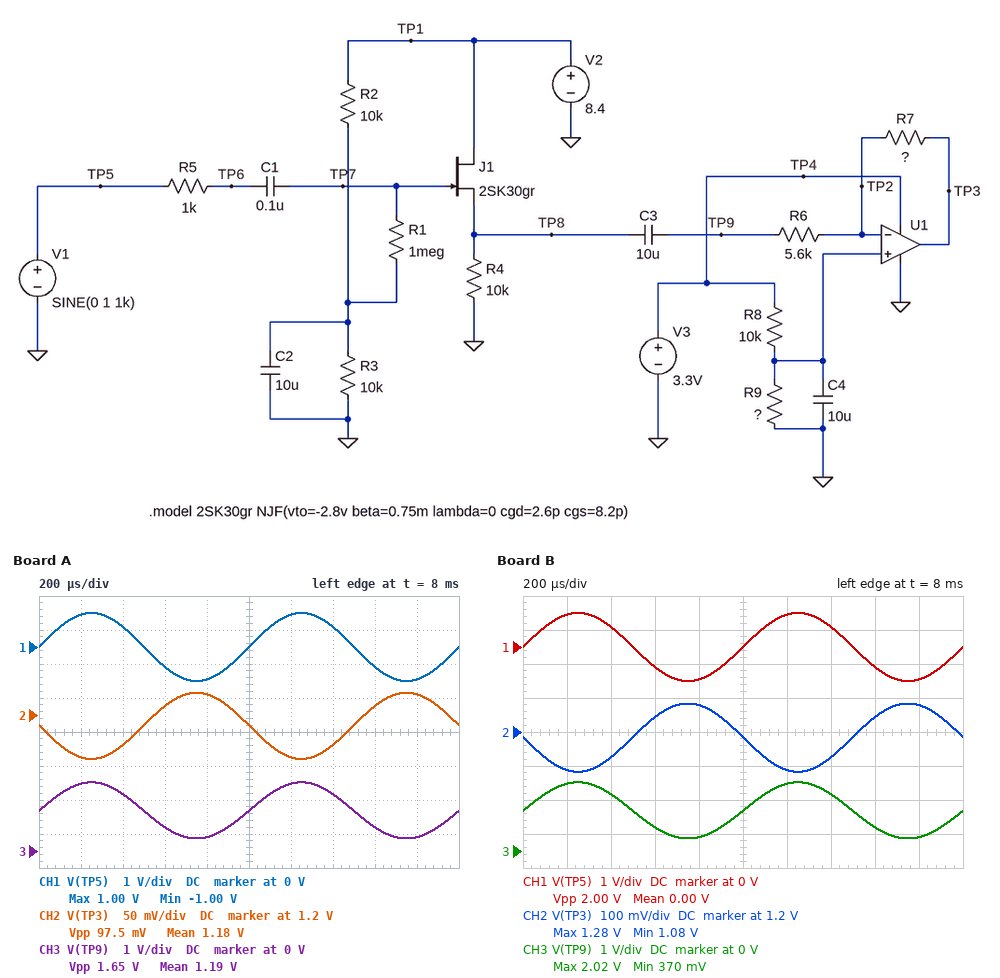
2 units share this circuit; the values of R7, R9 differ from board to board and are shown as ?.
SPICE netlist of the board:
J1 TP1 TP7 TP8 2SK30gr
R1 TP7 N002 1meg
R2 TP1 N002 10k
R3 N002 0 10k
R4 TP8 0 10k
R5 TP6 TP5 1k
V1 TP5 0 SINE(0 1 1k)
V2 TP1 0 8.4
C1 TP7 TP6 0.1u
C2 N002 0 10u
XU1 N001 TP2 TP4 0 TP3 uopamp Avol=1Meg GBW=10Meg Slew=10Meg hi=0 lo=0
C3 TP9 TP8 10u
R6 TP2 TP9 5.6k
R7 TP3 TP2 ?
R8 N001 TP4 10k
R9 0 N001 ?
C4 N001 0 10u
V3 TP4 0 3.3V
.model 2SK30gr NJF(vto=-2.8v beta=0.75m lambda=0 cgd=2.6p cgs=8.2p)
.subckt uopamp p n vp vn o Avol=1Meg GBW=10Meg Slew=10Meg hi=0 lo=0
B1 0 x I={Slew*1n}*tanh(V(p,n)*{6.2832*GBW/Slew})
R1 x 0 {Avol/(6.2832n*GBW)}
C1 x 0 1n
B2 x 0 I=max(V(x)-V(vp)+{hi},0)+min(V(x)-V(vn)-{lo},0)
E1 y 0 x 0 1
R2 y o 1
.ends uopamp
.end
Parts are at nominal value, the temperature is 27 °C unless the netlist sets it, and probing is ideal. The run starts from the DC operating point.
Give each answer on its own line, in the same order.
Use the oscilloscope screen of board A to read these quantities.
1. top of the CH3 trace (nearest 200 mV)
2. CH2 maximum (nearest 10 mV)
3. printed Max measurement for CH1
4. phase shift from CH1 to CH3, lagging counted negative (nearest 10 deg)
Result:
2.0 V
1.23 V
1.00 V
0 deg
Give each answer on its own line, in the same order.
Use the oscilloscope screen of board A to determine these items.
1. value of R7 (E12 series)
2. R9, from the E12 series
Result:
330 Ω
5.6 kΩ
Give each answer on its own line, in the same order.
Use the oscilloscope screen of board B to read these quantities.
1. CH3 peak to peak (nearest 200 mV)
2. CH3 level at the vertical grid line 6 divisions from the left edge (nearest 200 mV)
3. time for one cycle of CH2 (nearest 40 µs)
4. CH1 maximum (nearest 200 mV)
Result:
1.6 V
2.0 V
1.00 ms
1.0 V
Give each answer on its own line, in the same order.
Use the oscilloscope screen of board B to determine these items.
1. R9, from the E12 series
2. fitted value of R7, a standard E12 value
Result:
5.6 kΩ
680 Ω
